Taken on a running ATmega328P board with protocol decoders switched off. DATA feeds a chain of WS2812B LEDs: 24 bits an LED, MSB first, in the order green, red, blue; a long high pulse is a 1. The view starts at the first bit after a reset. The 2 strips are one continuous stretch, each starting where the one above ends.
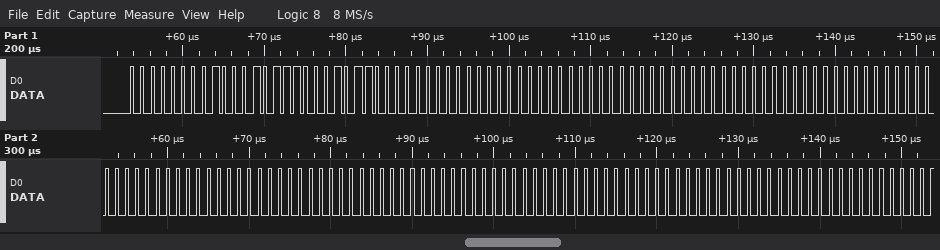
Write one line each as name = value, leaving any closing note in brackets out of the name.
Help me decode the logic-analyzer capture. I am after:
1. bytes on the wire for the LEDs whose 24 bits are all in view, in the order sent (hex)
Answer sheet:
bytes on the wire for the LEDs whose 24 bits are all in view, in the order sent = 00 8B 8B 00 00 00 00 00 00 00 00 00 00 00 00 00 00 00
